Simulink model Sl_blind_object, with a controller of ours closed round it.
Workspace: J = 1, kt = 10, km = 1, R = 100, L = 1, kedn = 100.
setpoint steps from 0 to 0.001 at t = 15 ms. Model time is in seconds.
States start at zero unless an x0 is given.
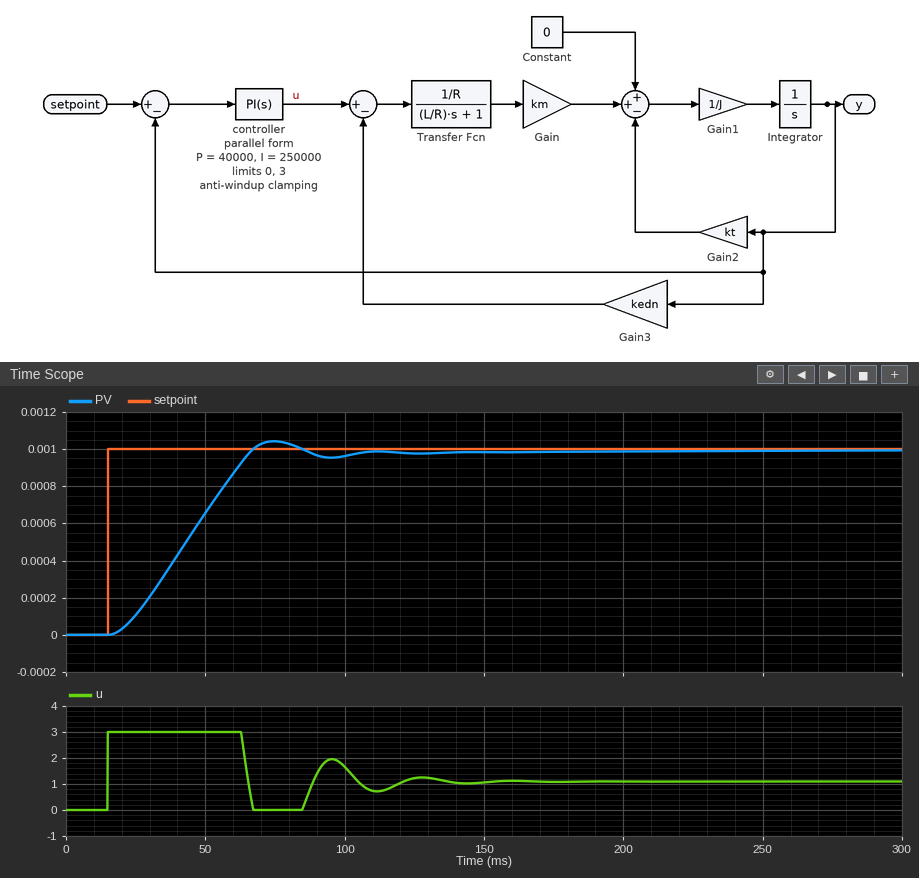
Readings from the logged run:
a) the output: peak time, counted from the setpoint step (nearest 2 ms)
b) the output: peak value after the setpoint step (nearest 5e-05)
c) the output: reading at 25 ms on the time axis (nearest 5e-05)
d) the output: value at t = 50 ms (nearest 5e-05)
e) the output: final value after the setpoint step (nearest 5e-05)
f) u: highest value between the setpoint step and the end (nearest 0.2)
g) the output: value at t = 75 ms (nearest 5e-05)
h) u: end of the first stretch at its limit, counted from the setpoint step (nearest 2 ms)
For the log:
60 ms
0.00105
0.00010
0.00065
0.00100
3.0
0.00105
48 ms
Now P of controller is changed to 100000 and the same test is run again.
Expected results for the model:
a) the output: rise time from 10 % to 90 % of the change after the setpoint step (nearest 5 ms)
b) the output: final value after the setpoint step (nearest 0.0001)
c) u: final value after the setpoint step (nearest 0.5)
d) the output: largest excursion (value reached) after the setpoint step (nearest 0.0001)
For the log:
35 ms
0.0010
1.0
0.0011
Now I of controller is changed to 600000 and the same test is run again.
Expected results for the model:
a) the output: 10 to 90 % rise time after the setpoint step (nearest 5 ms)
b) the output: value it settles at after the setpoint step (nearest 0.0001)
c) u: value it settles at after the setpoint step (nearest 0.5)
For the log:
35 ms
0.0010
1.0
